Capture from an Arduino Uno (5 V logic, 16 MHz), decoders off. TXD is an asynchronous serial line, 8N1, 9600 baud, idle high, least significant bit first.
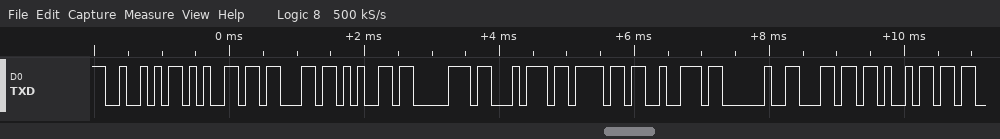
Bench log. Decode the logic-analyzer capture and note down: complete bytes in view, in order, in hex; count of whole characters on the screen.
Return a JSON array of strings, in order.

["0x52 0x65 0x63 0x65 0x70 0x74 0x6F 0x72 0x20 0x6C 0x69", "11"]
